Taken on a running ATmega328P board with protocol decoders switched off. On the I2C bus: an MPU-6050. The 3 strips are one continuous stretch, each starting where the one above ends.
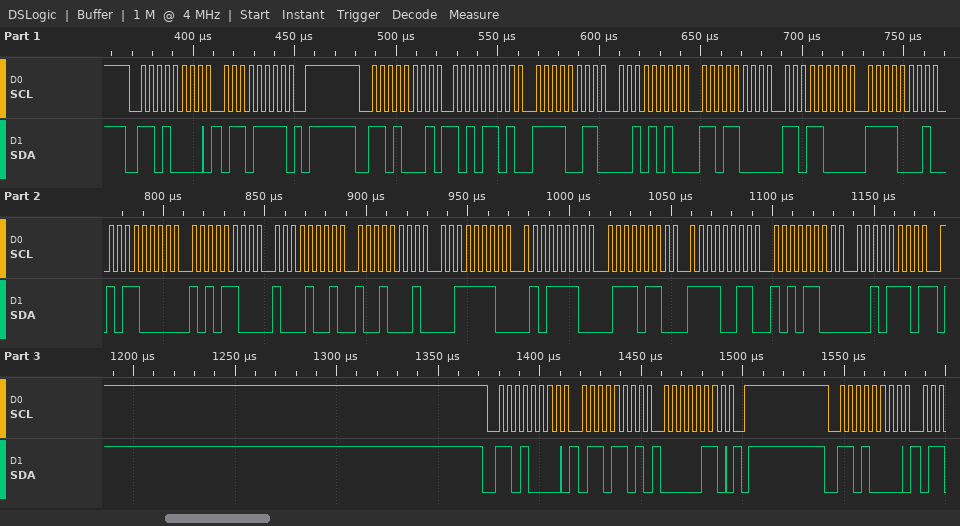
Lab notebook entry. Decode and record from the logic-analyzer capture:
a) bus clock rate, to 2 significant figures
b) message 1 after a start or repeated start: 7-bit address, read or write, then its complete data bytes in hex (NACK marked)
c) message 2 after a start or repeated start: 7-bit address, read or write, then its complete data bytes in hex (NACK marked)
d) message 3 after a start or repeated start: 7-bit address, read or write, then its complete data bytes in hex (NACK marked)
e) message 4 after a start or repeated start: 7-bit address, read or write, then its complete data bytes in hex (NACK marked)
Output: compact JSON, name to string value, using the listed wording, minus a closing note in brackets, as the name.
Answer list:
{"bus clock rate, to 2 significant figures": "250 kHz", "message 1 after a start or repeated start: 7-bit address, read or write, then its complete data bytes in hex": "0x68 write: 6F", "message 2 after a start or repeated start: 7-bit address, read or write, then its complete data bytes in hex": "0x68 read: AD F3 2A D8 D8 F1 B0 AC 89 91 3E 5E 76 F3 AC 2E NACK", "message 3 after a start or repeated start: 7-bit address, read or write, then its complete data bytes in hex": "0x68 write: 6D 06", "message 4 after a start or repeated start: 7-bit address, read or write, then its complete data bytes in hex": "0x68 write"}
